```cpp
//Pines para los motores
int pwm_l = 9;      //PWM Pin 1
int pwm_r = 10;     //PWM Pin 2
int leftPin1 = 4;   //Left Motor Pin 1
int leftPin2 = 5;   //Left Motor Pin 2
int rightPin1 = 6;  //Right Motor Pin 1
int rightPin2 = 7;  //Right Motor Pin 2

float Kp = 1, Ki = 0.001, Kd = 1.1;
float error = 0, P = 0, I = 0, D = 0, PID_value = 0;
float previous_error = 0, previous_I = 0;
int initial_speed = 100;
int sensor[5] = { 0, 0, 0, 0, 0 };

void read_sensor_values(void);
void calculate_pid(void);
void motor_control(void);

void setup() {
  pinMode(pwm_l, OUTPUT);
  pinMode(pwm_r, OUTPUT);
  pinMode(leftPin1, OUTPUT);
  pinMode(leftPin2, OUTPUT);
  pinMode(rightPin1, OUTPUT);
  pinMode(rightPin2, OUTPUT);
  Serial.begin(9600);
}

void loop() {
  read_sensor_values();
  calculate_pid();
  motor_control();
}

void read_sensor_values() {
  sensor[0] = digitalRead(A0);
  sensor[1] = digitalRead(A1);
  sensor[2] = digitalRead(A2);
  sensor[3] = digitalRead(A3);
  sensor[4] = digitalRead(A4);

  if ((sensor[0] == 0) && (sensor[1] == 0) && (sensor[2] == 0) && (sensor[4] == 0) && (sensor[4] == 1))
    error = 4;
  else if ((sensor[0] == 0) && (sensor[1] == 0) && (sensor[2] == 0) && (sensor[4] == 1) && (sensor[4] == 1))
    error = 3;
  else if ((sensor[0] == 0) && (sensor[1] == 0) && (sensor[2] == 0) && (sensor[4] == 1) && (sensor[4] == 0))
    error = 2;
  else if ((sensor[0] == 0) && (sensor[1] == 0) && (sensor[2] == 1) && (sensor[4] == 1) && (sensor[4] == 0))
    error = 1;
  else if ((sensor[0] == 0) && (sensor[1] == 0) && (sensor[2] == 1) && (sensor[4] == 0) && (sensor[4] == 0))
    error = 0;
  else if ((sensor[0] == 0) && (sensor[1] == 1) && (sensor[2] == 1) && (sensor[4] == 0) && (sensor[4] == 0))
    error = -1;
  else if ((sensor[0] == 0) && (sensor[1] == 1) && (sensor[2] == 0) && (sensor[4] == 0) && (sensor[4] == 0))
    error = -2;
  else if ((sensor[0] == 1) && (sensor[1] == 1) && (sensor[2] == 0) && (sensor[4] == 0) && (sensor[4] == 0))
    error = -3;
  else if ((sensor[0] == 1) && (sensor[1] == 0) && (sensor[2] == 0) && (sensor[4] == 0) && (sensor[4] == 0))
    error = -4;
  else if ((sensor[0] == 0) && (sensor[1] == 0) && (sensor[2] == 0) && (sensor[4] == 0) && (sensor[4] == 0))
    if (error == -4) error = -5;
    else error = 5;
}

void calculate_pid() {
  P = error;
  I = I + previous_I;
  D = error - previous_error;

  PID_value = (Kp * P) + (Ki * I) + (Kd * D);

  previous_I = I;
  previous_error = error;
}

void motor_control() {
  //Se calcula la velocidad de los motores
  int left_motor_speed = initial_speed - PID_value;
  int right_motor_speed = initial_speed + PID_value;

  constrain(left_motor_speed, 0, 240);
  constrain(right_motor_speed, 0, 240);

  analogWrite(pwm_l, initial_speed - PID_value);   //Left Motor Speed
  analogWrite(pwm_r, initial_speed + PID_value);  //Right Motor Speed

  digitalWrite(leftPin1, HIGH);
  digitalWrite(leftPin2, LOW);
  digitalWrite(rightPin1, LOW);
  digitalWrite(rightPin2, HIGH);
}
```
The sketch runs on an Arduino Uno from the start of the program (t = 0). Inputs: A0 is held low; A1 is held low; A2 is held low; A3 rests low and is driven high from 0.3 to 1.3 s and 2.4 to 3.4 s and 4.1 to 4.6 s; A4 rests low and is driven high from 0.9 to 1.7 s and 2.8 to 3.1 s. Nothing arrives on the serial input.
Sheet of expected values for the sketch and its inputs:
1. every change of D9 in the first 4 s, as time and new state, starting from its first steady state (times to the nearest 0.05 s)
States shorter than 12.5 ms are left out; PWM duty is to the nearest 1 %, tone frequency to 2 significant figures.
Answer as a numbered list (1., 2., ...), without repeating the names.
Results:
1. 0 s PWM 37 %; 0.9 s PWM 38 %; 1.7 s PWM 37 %; 2.8 s PWM 38 %; 3.1 s PWM 37 %
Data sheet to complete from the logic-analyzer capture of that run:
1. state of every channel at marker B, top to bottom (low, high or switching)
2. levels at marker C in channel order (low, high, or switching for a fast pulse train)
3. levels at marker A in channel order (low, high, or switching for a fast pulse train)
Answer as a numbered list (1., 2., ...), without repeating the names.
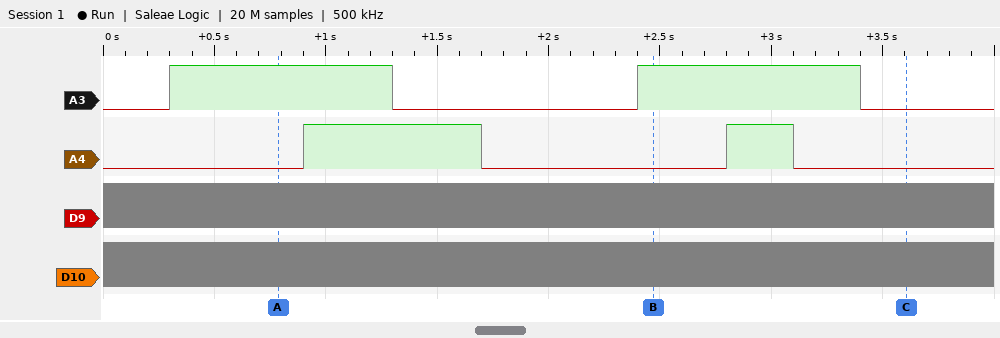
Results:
1. A3 high, A4 low, D9 switching, D10 switching
2. A3 low, A4 low, D9 switching, D10 switching
3. A3 high, A4 low, D9 switching, D10 switching
